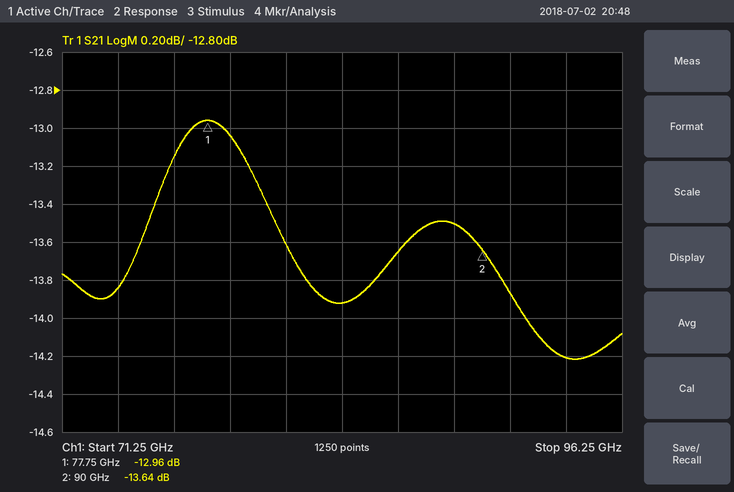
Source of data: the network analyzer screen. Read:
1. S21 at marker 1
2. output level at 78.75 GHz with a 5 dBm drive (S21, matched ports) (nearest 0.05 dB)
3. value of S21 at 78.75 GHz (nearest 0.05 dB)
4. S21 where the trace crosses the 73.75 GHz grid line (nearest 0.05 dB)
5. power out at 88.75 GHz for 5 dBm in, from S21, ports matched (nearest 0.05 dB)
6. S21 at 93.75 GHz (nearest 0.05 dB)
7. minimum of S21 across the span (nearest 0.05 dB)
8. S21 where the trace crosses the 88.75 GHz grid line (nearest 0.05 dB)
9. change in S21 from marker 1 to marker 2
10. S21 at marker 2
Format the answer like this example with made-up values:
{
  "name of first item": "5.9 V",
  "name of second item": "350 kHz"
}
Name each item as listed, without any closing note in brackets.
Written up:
{
  "S21 at marker 1": "-12.96 dB",
  "output level at 78.75 GHz with a 5 dBm drive (S21, matched ports)": "-8.05 dBm",
  "value of S21 at 78.75 GHz": "-13.05 dB",
  "S21 where the trace crosses the 73.75 GHz grid line": "-13.85 dB",
  "power out at 88.75 GHz for 5 dBm in, from S21, ports matched": "-8.50 dBm",
  "S21 at 93.75 GHz": "-14.20 dB",
  "minimum of S21 across the span": "-14.20 dB",
  "S21 where the trace crosses the 88.75 GHz grid line": "-13.50 dB",
  "change in S21 from marker 1 to marker 2": "-0.68 dB",
  "S21 at marker 2": "-13.64 dB"
}
